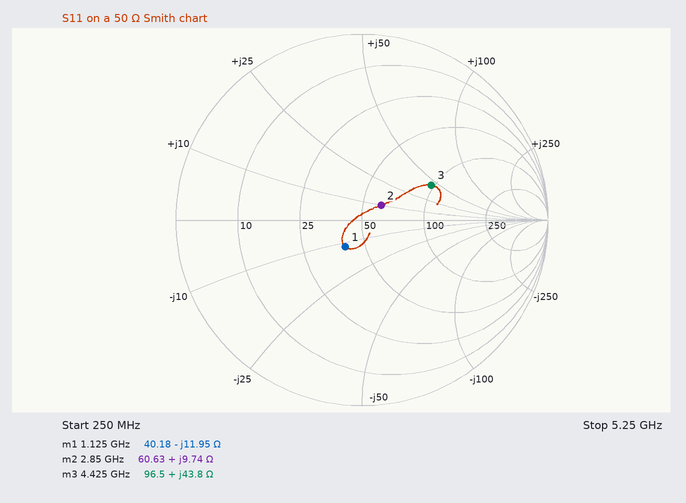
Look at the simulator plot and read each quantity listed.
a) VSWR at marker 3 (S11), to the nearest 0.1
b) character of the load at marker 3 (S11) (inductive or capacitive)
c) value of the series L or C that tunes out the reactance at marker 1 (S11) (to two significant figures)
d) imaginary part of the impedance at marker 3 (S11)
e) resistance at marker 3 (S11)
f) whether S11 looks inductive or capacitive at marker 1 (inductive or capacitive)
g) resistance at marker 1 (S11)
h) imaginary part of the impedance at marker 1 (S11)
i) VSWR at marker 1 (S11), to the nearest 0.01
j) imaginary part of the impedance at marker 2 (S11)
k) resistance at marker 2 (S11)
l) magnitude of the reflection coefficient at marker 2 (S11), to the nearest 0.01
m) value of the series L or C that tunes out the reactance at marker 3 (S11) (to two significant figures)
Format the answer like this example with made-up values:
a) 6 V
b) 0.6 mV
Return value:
a) 2.4
b) inductive
c) 1.7 nH
d) +43.8 Ω
e) 96.5 Ω
f) capacitive
g) 40.18 Ω
h) -11.95 Ω
i) 1.41
j) +9.74 Ω
k) 60.63 Ω
l) 0.13
m) 820 fF
